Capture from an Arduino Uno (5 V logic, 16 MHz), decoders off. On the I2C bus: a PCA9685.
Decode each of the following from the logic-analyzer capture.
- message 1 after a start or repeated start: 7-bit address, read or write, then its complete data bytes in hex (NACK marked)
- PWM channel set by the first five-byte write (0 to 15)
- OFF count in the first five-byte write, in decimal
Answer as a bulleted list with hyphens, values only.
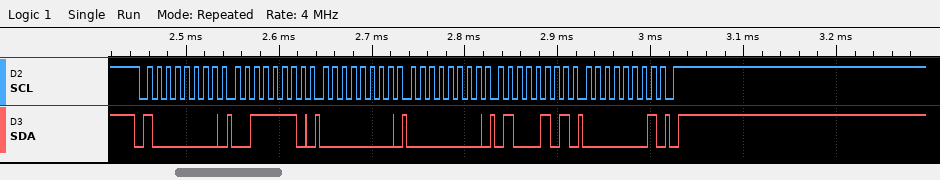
- 0x40 write: 3E 00 00 45 01
- 14
- 325
